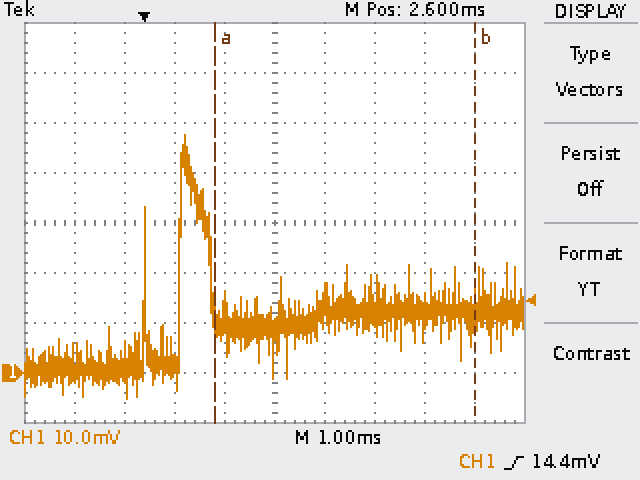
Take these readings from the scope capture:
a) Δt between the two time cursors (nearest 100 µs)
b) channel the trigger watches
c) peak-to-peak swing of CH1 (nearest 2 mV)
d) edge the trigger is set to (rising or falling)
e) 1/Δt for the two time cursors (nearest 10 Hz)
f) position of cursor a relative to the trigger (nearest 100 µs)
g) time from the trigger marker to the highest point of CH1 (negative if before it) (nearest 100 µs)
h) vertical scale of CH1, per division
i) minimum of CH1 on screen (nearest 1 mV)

5.2 ms
CH1
52 mV
rising
190 Hz
+1.4 ms
+800 µs
10 mV
-5 mV
